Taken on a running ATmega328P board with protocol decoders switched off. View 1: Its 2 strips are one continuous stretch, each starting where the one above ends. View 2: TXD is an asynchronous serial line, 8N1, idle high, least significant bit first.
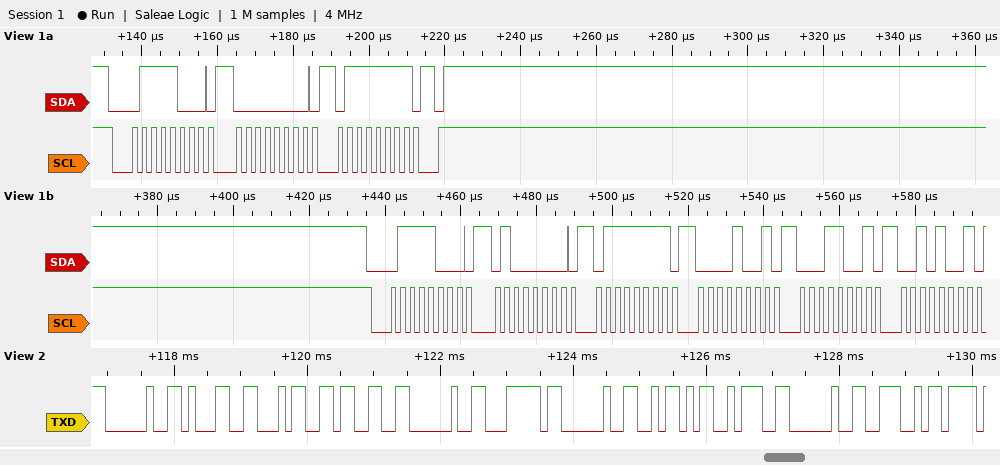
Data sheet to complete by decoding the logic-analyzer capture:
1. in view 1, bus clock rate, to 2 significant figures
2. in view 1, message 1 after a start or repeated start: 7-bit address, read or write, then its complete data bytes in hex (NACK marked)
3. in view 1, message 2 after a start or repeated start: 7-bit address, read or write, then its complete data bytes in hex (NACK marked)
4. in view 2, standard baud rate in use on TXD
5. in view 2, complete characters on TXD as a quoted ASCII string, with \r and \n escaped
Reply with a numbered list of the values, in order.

1. 400 kHz
2. 0x3C write: 00 7F
3. 0x3C write: 40 7F 09 19 29
4. 9600 baud
5. " 143 | Z: N"
